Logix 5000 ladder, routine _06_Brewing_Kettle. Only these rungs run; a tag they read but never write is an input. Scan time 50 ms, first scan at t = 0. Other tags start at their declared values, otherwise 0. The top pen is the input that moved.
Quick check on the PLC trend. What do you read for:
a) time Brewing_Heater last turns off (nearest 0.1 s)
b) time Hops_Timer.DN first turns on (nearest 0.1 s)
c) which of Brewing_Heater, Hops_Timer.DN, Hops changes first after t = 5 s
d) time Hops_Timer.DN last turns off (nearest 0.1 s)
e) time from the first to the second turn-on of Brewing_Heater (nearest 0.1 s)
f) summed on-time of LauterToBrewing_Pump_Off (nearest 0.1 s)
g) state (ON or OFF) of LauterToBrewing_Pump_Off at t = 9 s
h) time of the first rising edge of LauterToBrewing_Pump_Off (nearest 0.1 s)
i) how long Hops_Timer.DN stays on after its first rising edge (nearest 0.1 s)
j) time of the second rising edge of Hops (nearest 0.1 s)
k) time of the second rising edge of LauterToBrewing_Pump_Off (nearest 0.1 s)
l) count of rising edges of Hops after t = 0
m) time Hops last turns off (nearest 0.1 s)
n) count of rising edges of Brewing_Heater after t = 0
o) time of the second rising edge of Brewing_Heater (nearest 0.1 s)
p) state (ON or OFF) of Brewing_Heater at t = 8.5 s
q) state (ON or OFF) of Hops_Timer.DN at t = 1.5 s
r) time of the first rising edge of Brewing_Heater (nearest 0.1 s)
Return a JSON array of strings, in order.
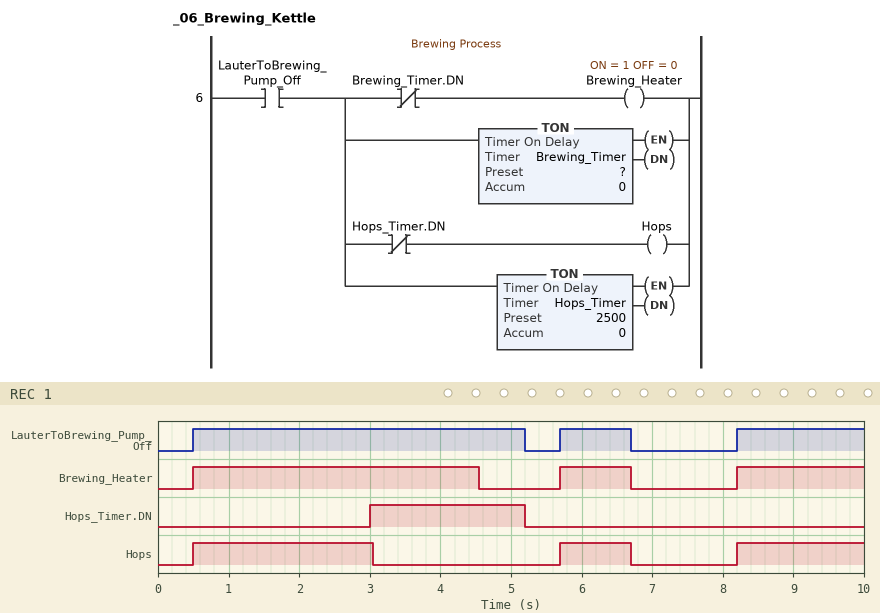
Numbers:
["6.7 s", "3.0 s", "Hops_Timer.DN", "5.2 s", "5.2 s", "7.5 s", "ON", "0.5 s", "2.2 s", "5.7 s", "5.7 s", "3", "6.7 s", "3", "5.7 s", "ON", "OFF", "0.5 s"]
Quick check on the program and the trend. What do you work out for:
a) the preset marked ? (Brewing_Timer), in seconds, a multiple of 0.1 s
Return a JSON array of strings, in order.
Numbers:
["4.0 s"]
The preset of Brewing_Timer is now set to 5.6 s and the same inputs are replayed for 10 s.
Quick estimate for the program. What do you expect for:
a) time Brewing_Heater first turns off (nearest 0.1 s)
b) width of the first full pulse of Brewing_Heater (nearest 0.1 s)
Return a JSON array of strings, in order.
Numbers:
["5.2 s", "4.7 s"]
